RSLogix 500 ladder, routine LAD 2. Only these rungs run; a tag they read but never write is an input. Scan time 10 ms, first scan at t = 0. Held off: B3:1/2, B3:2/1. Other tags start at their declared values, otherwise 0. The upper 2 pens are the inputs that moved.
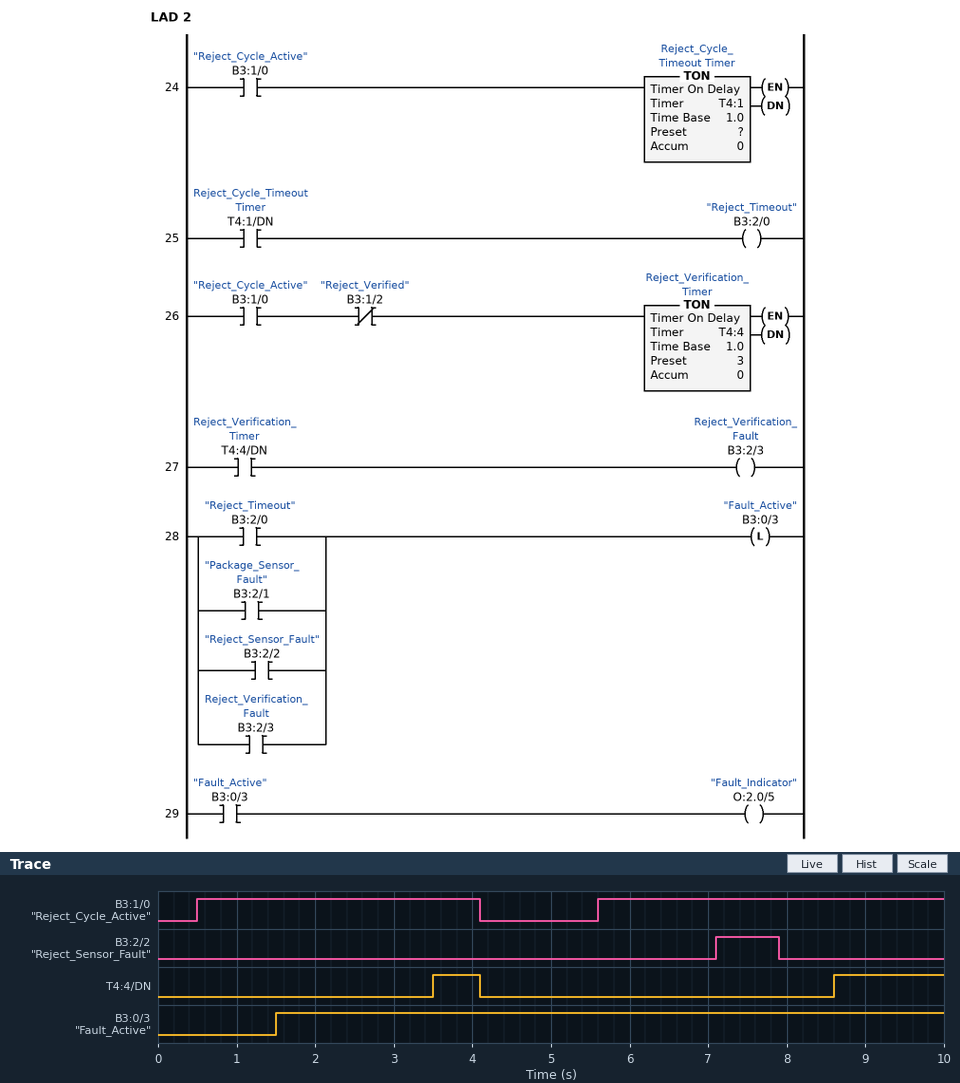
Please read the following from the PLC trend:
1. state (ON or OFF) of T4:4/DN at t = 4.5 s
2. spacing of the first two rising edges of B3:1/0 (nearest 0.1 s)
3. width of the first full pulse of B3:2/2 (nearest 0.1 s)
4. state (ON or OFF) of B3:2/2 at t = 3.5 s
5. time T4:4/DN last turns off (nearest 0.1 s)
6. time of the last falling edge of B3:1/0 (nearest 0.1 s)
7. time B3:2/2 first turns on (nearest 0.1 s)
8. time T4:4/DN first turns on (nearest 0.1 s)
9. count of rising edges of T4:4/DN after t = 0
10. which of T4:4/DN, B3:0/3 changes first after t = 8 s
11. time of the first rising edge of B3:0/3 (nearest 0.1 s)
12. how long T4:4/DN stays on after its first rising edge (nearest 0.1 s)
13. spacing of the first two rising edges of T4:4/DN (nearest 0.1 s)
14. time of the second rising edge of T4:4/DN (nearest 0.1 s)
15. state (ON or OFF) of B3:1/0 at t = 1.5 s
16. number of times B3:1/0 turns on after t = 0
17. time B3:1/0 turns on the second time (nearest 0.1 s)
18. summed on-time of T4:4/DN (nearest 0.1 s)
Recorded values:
OFF
5.1 s
0.8 s
OFF
4.1 s
4.1 s
7.1 s
3.5 s
2
T4:4/DN
1.5 s
0.6 s
5.1 s
8.6 s
ON
2
5.6 s
2.0 s
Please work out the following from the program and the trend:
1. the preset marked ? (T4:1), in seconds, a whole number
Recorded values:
1 s
